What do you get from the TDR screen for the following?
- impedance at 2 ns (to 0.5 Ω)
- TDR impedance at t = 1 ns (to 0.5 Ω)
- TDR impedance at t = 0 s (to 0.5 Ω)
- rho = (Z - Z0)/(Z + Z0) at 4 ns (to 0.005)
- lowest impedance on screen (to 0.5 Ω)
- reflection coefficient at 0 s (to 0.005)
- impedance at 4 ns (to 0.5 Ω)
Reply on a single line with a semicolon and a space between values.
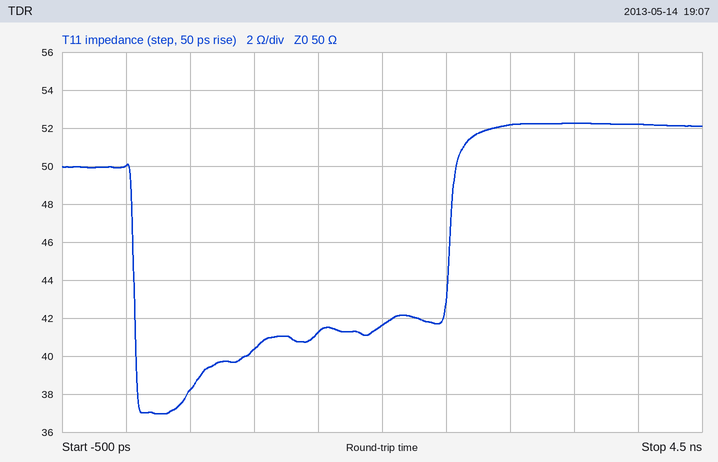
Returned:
41.5 Ω; 40.5 Ω; 50.0 Ω; +0.020; 37.0 Ω; 0.000; 52.0 Ω
